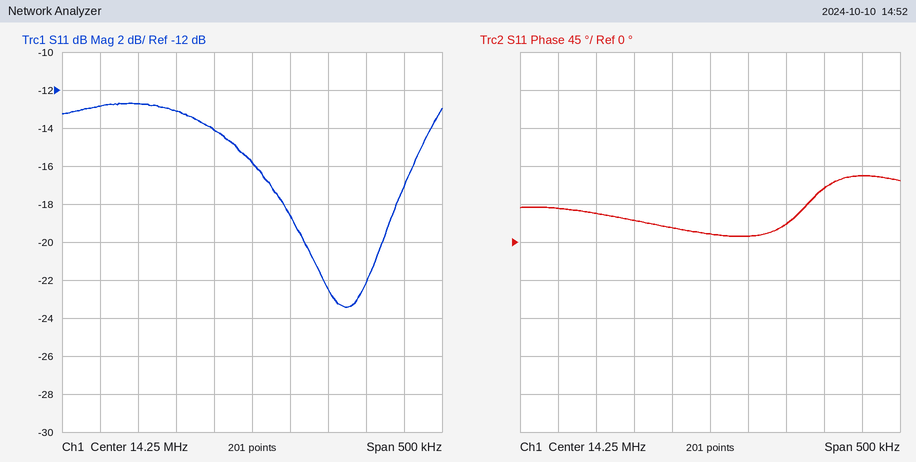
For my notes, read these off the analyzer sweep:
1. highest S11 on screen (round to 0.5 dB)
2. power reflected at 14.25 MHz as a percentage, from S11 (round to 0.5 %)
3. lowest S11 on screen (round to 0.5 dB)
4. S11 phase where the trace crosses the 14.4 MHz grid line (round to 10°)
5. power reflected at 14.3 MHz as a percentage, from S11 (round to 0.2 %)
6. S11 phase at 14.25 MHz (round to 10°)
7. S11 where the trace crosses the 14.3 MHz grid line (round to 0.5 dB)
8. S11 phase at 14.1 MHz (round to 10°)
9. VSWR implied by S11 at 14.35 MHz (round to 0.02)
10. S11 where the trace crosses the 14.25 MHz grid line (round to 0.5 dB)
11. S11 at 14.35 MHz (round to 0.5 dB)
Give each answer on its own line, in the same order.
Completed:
-12.5 dB
2.5 %
-23.5 dB
60°
1.4 %
10°
-18.5 dB
30°
1.16
-16.0 dB
-22.5 dB
